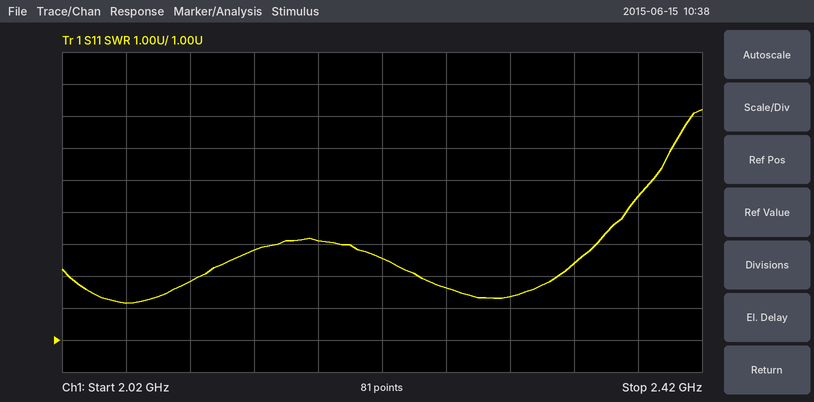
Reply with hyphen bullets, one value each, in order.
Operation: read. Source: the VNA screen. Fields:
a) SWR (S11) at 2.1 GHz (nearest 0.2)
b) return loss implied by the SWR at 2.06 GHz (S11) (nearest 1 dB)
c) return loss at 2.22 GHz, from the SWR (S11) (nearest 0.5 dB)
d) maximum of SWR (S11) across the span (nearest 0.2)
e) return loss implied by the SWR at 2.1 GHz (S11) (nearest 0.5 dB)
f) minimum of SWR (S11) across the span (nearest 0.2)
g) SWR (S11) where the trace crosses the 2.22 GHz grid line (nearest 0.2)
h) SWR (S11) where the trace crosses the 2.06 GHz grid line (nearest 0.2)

- 2.8
- 9 dB
- 5.0 dB
- 8.2
- 6.5 dB
- 2.2
- 3.6
- 2.2
